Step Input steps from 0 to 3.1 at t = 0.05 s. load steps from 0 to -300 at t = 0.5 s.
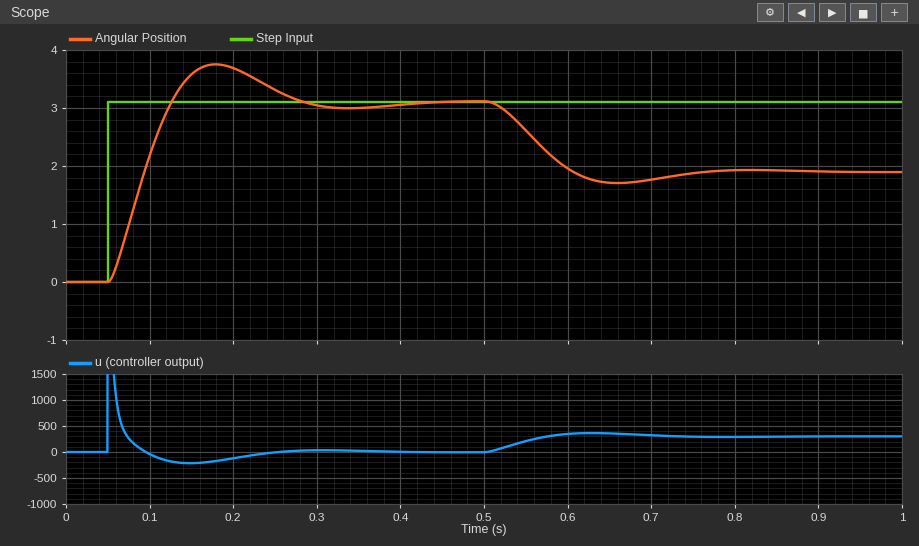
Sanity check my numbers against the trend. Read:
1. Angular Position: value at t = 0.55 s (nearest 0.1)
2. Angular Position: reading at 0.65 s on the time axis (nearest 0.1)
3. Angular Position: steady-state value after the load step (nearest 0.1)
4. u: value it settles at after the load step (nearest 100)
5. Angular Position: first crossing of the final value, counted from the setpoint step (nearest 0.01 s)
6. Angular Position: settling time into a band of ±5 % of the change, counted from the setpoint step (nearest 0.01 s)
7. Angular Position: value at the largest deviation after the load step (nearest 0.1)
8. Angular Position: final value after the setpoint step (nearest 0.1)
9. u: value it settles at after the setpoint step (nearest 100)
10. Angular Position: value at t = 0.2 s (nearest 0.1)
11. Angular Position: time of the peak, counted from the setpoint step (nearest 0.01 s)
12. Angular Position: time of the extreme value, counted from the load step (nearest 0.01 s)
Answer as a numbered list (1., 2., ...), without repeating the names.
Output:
1. 2.6
2. 1.7
3. 1.9
4. 300
5. 0.08 s
6. 0.21 s
7. 1.7
8. 3.1
9. 0
10. 3.7
11. 0.13 s
12. 0.16 s
